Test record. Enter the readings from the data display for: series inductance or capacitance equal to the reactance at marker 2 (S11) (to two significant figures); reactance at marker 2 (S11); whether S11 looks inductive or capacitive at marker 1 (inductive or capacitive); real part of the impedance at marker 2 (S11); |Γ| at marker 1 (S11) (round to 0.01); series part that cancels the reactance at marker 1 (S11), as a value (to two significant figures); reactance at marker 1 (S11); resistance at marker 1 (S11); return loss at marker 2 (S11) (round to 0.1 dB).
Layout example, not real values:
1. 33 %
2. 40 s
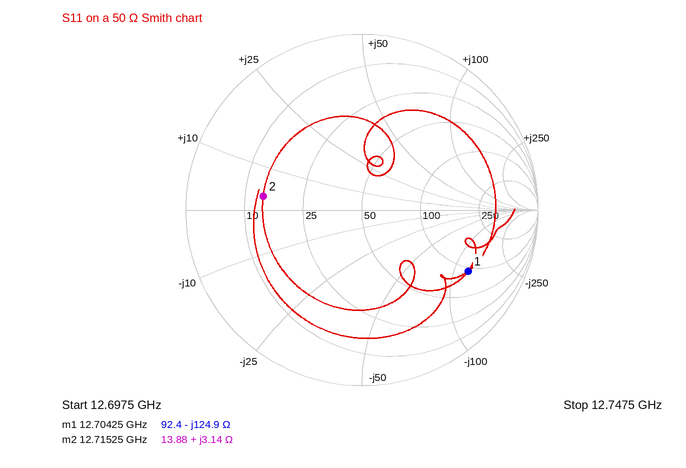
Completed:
1. 39 pH
2. +3.14 Ω
3. capacitive
4. 13.88 Ω
5. 0.70
6. 1.6 nH
7. -124.9 Ω
8. 92.4 Ω
9. 4.9 dB
